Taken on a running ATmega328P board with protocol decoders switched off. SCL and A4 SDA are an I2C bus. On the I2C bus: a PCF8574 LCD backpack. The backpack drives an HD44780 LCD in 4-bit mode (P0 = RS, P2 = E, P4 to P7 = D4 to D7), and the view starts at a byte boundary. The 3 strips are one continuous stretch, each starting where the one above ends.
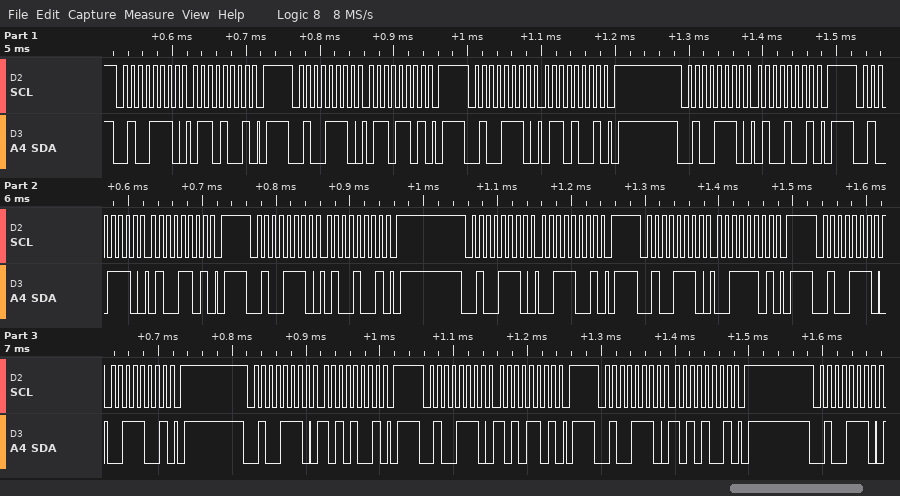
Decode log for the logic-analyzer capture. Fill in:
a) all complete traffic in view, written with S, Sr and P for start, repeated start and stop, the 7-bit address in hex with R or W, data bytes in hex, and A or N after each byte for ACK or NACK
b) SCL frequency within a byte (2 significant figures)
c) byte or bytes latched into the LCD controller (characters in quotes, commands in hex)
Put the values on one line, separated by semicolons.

S 27W A 69 A P S 27W A 6D A P S 27W A 69 A P S 27W A 49 A P S 27W A 4D A P S 27W A 49 A P S 27W A 39 A P S 27W A 3D A P S 27W A 39 A P S 27W A A9 A P S 27W A AD A P S 27W A A9 A P S 27W A; 100 kHz; 'd' ':'
